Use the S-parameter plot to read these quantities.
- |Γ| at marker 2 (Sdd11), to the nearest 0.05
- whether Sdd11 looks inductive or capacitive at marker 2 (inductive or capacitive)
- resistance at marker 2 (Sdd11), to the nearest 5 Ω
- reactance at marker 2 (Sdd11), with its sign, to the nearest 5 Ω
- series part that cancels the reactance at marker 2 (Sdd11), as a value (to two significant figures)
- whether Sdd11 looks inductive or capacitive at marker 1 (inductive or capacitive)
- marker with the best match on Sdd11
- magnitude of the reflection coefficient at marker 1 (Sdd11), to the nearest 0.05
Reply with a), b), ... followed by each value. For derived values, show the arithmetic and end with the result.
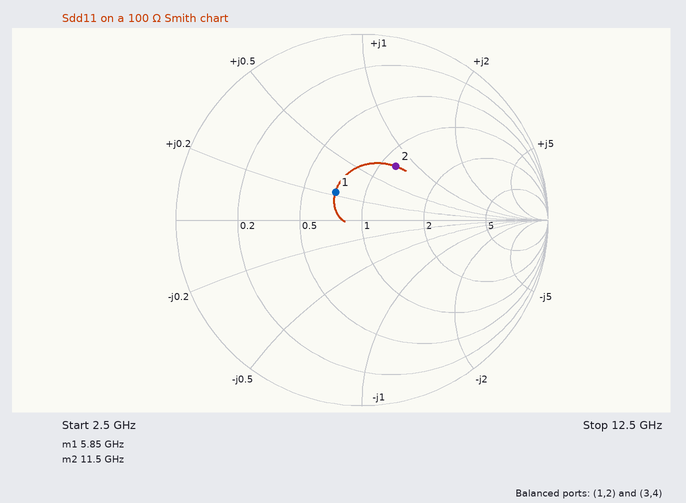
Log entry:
a) 0.35
b) inductive
c) 115 Ω
d) +75 Ω
e) C = 1/(2π × 11.5 GHz × 75 Ω) ≈ 185 fF, so 180 fF to two significant figures
f) inductive
g) marker 1
h) 0.20
